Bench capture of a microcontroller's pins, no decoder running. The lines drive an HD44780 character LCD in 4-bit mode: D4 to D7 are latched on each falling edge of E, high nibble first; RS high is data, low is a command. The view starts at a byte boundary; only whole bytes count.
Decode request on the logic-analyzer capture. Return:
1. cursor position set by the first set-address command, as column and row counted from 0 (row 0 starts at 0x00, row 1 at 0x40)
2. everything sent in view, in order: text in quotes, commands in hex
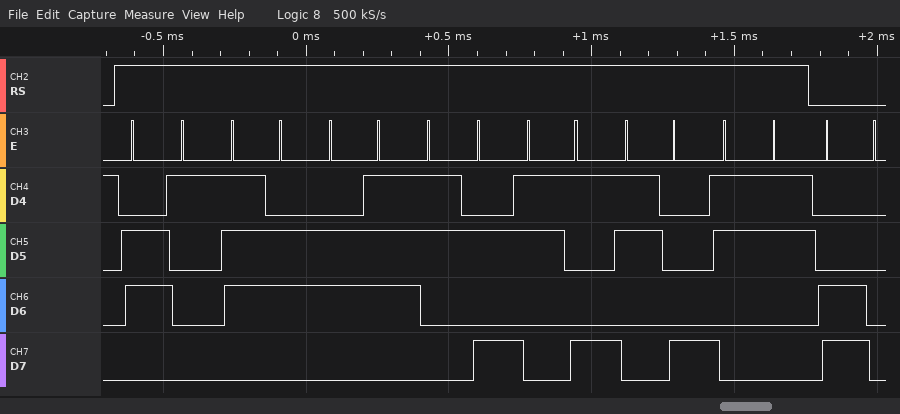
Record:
column 0, row 1
"avg:983" 0xC0
